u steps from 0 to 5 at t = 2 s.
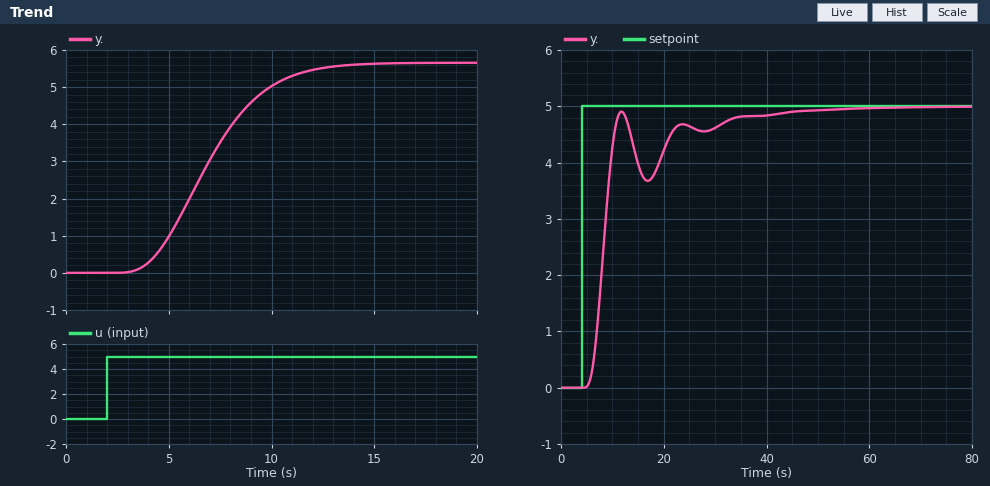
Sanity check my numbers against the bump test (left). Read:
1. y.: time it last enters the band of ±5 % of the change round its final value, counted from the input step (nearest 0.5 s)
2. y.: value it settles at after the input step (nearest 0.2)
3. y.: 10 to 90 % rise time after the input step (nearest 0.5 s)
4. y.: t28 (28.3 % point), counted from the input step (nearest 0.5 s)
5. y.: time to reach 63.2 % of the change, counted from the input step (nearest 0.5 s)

9.5 s
5.6
5.5 s
3.5 s
5.5 s
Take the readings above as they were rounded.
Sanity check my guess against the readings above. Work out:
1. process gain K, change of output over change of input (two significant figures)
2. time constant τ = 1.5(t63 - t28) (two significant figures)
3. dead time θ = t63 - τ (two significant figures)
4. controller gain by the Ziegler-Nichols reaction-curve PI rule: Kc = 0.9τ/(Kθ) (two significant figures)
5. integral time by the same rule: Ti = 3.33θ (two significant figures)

1.1
3.0 s
2.5 s
0.98
8.3 s
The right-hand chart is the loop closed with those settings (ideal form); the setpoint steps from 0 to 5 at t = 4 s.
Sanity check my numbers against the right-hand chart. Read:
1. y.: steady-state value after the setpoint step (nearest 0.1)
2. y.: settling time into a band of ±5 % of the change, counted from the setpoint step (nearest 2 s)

5.0
28 s
